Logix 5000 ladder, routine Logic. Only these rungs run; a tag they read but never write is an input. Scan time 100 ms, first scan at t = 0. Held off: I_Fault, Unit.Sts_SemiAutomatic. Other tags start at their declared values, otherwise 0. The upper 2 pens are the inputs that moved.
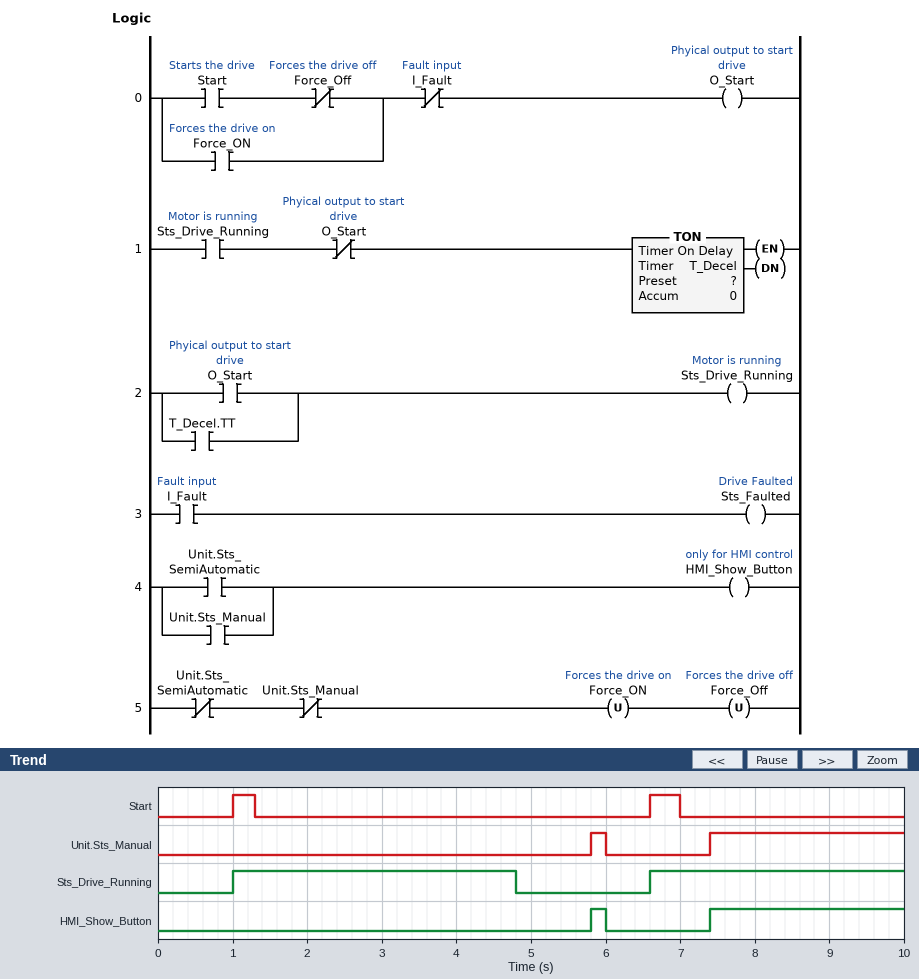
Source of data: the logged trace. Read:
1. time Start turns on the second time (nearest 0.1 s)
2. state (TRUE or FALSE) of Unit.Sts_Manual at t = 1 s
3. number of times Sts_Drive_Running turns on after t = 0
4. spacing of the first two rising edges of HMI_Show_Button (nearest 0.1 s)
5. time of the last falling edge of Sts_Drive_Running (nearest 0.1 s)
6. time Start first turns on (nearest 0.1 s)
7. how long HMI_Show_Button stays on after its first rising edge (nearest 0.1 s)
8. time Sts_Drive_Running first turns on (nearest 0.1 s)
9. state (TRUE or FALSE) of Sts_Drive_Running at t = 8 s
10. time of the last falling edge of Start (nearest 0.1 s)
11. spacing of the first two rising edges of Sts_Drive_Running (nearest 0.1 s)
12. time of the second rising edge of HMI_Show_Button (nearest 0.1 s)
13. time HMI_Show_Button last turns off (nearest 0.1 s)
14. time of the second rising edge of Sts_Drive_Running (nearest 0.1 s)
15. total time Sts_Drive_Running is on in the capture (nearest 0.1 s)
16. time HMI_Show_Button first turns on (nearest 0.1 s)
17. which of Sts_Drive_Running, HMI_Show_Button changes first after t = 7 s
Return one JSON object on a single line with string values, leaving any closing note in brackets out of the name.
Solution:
{"time Start turns on the second time": "6.6 s", "state (TRUE or FALSE) of Unit.Sts_Manual at t = 1 s": "FALSE", "number of times Sts_Drive_Running turns on after t = 0": "2", "spacing of the first two rising edges of HMI_Show_Button": "1.6 s", "time of the last falling edge of Sts_Drive_Running": "4.8 s", "time Start first turns on": "1.0 s", "how long HMI_Show_Button stays on after its first rising edge": "0.2 s", "time Sts_Drive_Running first turns on": "1.0 s", "state (TRUE or FALSE) of Sts_Drive_Running at t = 8 s": "TRUE", "time of the last falling edge of Start": "7.0 s", "spacing of the first two rising edges of Sts_Drive_Running": "5.6 s", "time of the second rising edge of HMI_Show_Button": "7.4 s", "time HMI_Show_Button last turns off": "6.0 s", "time of the second rising edge of Sts_Drive_Running": "6.6 s", "total time Sts_Drive_Running is on in the capture": "7.2 s", "time HMI_Show_Button first turns on": "5.8 s", "which of Sts_Drive_Running, HMI_Show_Button changes first after t = 7 s": "HMI_Show_Button"}
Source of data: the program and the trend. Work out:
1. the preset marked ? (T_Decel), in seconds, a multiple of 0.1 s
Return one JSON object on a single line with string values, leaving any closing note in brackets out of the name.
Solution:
{"the preset marked ? (T_Decel), in seconds, a multiple of 0.1 s": "3.5 s"}
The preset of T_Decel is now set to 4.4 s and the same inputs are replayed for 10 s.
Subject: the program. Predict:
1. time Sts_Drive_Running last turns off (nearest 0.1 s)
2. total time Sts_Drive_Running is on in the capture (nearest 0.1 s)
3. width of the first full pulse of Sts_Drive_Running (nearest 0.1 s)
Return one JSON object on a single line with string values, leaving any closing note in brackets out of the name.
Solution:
{"time Sts_Drive_Running last turns off": "5.7 s", "total time Sts_Drive_Running is on in the capture": "8.1 s", "width of the first full pulse of Sts_Drive_Running": "4.7 s"}
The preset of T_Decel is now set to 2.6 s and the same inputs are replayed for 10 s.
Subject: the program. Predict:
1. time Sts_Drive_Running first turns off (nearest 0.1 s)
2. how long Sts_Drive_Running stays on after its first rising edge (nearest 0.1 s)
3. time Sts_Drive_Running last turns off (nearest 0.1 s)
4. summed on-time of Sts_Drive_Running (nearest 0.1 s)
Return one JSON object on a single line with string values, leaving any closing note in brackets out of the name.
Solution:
{"time Sts_Drive_Running first turns off": "3.9 s", "how long Sts_Drive_Running stays on after its first rising edge": "2.9 s", "time Sts_Drive_Running last turns off": "9.6 s", "summed on-time of Sts_Drive_Running": "5.9 s"}
